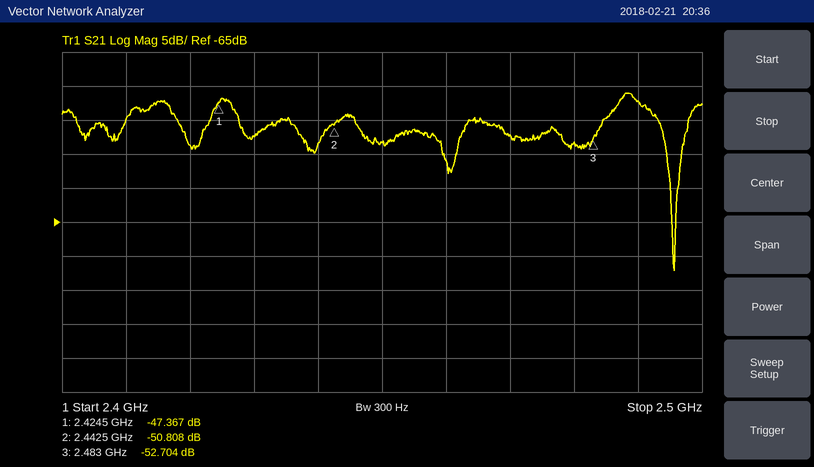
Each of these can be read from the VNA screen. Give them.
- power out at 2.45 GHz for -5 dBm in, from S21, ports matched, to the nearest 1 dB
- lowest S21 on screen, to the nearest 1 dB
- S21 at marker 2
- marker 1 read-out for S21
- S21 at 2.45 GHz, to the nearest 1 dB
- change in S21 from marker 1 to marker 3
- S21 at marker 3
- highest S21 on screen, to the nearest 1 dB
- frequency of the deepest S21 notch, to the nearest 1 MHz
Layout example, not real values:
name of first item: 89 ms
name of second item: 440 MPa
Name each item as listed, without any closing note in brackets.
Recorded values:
power out at 2.45 GHz for -5 dBm in, from S21, ports matched, to the nearest 1 dB: -58 dBm
lowest S21 on screen, to the nearest 1 dB: -72 dB
S21 at marker 2: -50.808 dB
marker 1 read-out for S21: -47.367 dB
S21 at 2.45 GHz, to the nearest 1 dB: -53 dB
change in S21 from marker 1 to marker 3: -5.337 dB
S21 at marker 3: -52.704 dB
highest S21 on screen, to the nearest 1 dB: -46 dB
frequency of the deepest S21 notch, to the nearest 1 MHz: 2.496 GHz
